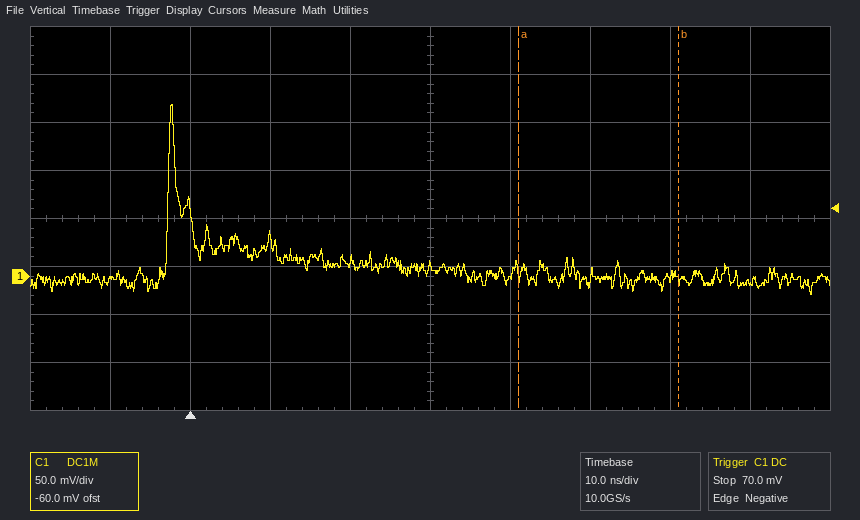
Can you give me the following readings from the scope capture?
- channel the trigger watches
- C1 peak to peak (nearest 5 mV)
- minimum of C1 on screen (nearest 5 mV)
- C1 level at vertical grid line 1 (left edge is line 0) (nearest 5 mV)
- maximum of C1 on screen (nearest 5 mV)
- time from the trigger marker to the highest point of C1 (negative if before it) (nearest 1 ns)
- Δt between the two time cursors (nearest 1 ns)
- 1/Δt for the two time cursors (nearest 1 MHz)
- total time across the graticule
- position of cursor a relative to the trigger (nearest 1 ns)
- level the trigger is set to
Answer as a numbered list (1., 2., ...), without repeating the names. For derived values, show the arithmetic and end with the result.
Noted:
1. C1
2. 180 mV − (-20 mV) = 200 mV
3. -20 mV
4. -5 mV
5. 180 mV
6. -2 ns
7. 20 ns
8. 1 / 20 ns ≈ 50 MHz
9. 100 ns
10. +41 ns
11. 70.0 mV
